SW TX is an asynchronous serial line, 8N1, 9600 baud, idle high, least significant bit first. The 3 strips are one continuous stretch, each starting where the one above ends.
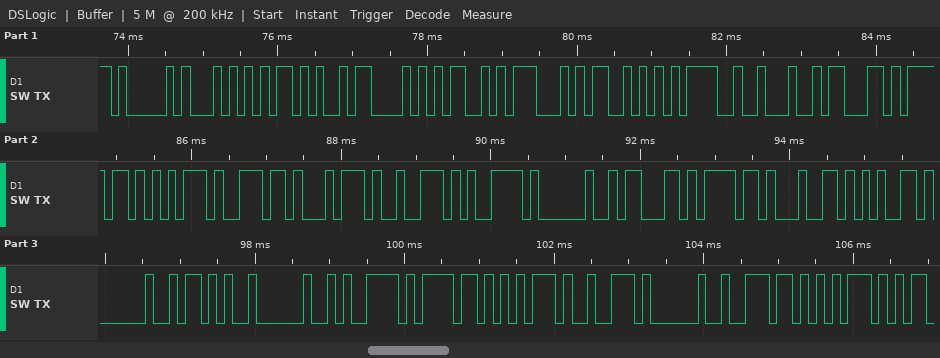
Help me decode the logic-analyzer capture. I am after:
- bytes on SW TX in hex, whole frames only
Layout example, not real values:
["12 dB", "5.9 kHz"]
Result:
["41 54 2B 43 4D 47 53 3D 22 63 6F 75 6E 74 72 79 20 63 6F 64 65 20 2B 20 79 6F 75 72 20 6E 75"]
